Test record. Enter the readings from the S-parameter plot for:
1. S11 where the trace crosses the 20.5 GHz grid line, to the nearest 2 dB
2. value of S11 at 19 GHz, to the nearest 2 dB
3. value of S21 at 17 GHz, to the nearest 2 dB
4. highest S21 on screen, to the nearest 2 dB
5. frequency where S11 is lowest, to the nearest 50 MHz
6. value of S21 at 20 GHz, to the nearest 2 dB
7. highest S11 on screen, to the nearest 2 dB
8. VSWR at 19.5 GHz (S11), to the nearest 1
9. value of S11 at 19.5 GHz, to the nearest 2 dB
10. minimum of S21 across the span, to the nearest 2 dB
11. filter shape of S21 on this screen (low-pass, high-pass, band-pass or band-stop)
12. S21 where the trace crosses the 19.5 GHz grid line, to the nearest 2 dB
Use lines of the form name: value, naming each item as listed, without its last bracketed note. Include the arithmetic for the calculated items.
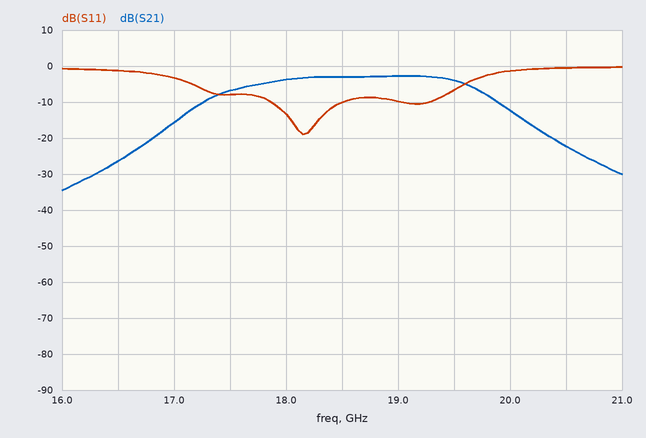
S11 where the trace crosses the 20.5 GHz grid line, to the nearest 2 dB: 0 dB
value of S11 at 19 GHz, to the nearest 2 dB: -10 dB
value of S21 at 17 GHz, to the nearest 2 dB: -16 dB
highest S21 on screen, to the nearest 2 dB: -2 dB
frequency where S11 is lowest, to the nearest 50 MHz: 18.15 GHz
value of S21 at 20 GHz, to the nearest 2 dB: -12 dB
highest S11 on screen, to the nearest 2 dB: 0 dB
VSWR at 19.5 GHz (S11), to the nearest 1: |Γ| = 10^(-6/20) = 0.5012; VSWR = (1 + 0.5012)/(1 − 0.5012) ≈ 3
value of S11 at 19.5 GHz, to the nearest 2 dB: -6 dB
minimum of S21 across the span, to the nearest 2 dB: -34 dB
filter shape of S21 on this screen: band-pass
S21 where the trace crosses the 19.5 GHz grid line, to the nearest 2 dB: -4 dB
